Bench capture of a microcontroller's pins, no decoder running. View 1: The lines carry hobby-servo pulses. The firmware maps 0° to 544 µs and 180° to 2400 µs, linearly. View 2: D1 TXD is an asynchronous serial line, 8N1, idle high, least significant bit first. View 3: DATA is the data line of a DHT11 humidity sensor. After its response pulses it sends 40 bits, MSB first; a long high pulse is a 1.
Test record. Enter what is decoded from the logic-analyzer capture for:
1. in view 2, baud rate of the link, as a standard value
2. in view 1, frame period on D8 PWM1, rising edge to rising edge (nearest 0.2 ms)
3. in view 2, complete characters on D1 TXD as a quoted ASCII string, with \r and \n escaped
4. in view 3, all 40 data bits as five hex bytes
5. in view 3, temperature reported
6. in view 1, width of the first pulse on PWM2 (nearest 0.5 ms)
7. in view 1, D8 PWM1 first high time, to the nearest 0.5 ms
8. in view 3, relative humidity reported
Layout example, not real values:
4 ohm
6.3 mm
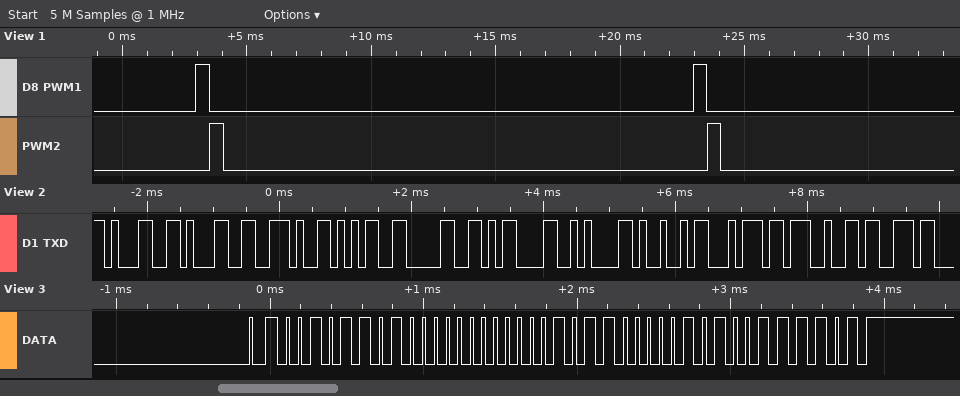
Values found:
9600 baud
20.0 ms
"11.50\r\nIt's"
2D 00 0B 05 3D
11.5 °C
0.5 ms
0.5 ms
45 %
